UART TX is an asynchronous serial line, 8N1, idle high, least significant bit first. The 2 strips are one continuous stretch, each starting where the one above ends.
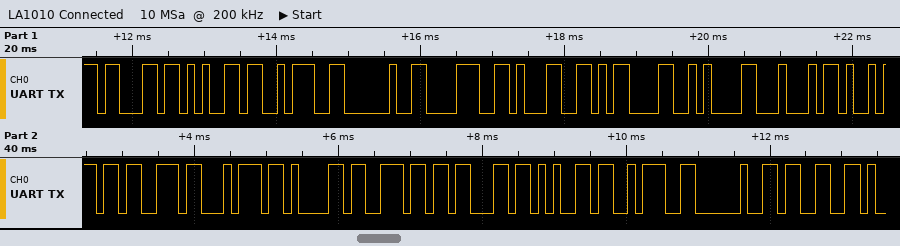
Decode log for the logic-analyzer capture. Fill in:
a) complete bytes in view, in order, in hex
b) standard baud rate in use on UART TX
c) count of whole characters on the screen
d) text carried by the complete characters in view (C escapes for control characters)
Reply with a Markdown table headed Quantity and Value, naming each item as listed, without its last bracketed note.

| Quantity | Value |
|---|---|
| complete bytes in view, in order, in hex | 0x63 0x65 0x3A 0x20 0x38 0x31 0x0D 0x0A 0x44 0x69 0x73 0x74 0x61 0x6E 0x63 0x65 0x3A 0x20 0x33 |
| standard baud rate in use on UART TX | 9600 baud |
| count of whole characters on the screen | 19 |
| text carried by the complete characters in view | "ce: 81\r\nDistance: 3" |
